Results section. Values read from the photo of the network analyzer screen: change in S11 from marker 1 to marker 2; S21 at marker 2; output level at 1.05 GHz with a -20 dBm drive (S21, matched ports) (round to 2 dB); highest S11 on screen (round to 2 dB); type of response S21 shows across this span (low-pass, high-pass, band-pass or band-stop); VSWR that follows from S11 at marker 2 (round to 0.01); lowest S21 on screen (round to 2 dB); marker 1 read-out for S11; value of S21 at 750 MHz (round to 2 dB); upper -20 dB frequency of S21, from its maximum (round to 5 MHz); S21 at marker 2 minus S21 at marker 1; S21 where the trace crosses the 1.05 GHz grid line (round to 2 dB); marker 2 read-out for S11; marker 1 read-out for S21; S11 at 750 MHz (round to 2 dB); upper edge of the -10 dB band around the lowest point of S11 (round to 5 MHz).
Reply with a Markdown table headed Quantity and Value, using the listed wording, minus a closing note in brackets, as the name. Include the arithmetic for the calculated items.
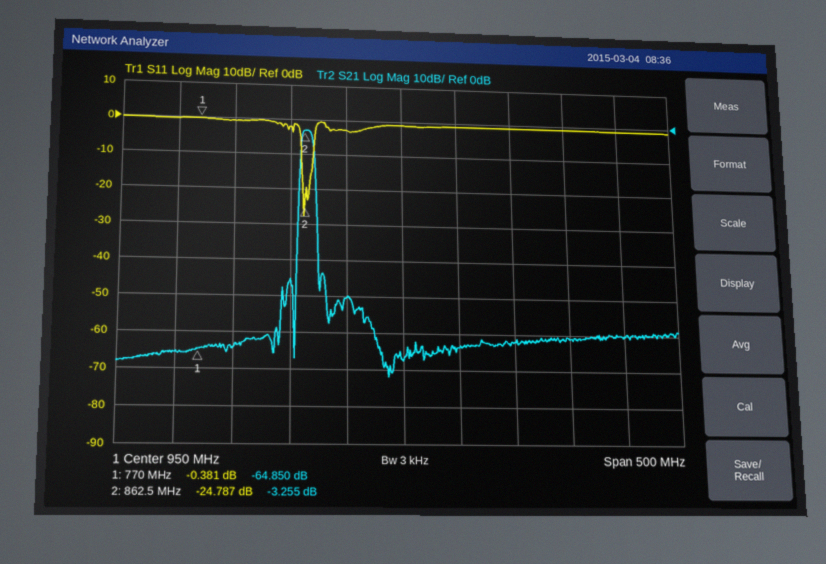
| Quantity | Value |
|---|---|
| change in S11 from marker 1 to marker 2 | -24.787 − (-0.381) = -24.406 dB |
| S21 at marker 2 | -3.255 dB |
| output level at 1.05 GHz with a -20 dBm drive (S21, matched ports) | -20 dBm + (-62 dB) = -82 dBm |
| highest S11 on screen | 0 dB |
| type of response S21 shows across this span | band-pass |
| VSWR that follows from S11 at marker 2 | (1 + 0.0576)/(1 − 0.0576) ≈ 1.12 |
| lowest S21 on screen | -72 dB |
| marker 1 read-out for S11 | -0.381 dB |
| value of S21 at 750 MHz | -66 dB |
| upper -20 dB frequency of S21, from its maximum | 875 MHz |
| S21 at marker 2 minus S21 at marker 1 | -3.255 − (-64.85) = 61.595 dB |
| S21 where the trace crosses the 1.05 GHz grid line | -62 dB |
| marker 2 read-out for S11 | -24.787 dB |
| marker 1 read-out for S21 | -64.850 dB |
| S11 at 750 MHz | 0 dB |
| upper edge of the -10 dB band around the lowest point of S11 | 870 MHz |
